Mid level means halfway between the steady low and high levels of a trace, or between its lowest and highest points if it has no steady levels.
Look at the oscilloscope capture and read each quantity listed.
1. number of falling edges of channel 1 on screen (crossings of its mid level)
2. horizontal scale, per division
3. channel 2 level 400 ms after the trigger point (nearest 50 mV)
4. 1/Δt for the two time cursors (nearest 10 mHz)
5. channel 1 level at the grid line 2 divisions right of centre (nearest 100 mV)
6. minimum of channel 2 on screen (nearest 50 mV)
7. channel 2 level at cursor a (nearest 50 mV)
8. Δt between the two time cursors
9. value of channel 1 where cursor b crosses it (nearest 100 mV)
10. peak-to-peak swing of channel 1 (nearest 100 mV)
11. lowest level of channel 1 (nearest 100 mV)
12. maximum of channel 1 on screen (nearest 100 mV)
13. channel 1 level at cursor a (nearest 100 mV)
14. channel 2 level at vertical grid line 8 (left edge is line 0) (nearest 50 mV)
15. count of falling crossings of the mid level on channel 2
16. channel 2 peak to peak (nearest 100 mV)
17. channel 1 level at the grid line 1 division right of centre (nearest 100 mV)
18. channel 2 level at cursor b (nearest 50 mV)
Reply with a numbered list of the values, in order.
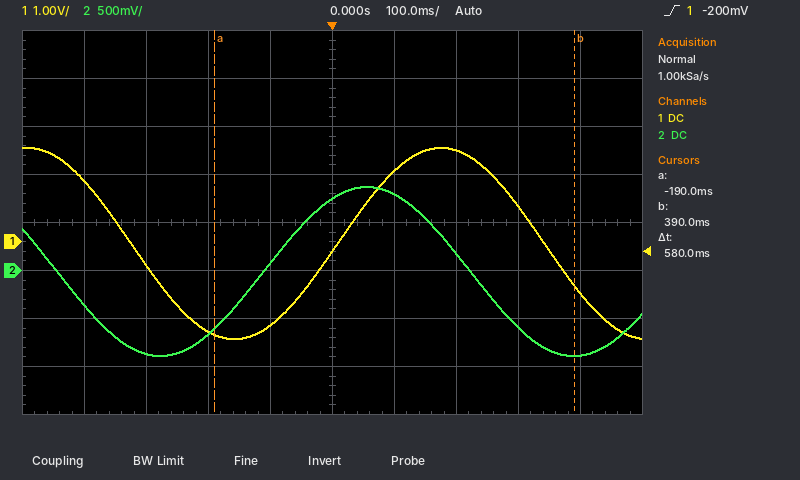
1. 2
2. 100 ms
3. -900 mV
4. 1.72 Hz
5. 1.9 V
6. -900 mV
7. -600 mV
8. 580 ms
9. -900 mV
10. 4.0 V
11. -2.0 V
12. 2.0 V
13. -1.9 V
14. -600 mV
15. 2
16. 1.80 V
17. 1.5 V
18. -900 mV
